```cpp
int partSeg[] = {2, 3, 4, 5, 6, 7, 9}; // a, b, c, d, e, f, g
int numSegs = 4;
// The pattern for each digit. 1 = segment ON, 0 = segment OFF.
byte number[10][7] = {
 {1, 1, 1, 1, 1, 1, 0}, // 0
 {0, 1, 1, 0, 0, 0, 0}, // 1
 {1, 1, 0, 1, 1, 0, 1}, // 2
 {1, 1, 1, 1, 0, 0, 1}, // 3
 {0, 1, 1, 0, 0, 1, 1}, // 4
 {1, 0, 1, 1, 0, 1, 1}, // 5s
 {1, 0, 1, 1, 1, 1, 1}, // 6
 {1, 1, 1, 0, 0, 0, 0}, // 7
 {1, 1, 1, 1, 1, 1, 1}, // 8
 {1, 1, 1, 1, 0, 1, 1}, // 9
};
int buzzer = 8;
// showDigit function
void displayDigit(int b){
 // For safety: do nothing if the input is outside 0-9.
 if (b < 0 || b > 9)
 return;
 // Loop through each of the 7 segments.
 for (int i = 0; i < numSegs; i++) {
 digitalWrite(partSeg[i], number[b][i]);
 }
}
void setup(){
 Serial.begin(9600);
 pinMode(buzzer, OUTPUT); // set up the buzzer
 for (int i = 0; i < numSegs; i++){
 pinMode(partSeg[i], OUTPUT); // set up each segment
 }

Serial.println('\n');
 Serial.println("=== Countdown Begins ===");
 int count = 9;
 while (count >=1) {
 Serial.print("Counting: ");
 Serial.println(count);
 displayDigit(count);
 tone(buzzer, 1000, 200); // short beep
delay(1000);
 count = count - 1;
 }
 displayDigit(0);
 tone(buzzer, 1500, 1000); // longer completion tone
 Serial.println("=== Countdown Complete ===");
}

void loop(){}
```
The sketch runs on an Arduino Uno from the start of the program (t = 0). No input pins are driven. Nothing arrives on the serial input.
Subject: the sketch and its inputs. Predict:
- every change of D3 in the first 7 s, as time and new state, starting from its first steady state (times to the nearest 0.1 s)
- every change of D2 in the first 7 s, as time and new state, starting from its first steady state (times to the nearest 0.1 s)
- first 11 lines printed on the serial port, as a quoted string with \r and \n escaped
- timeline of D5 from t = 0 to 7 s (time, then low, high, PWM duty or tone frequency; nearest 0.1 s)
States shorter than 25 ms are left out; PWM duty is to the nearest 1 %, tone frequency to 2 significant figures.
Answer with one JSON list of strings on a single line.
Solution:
["0 s high; 3 s low; 5 s high", "0 s high; 5 s low; 6 s high", "\"\\n\\r\\n=== Countdown Begins ===\\r\\nCounting: 9\\r\\nCounting: 8\\r\\nCounting: 7\\r\\nCounting: 6\\r\\nCounting: 5\\r\\nCounting: 4\\r\\nCounting: 3\\r\\nCounting: 2\\r\\n\"", "0 s high; 2 s low; 3 s high; 5 s low; 6 s high"]
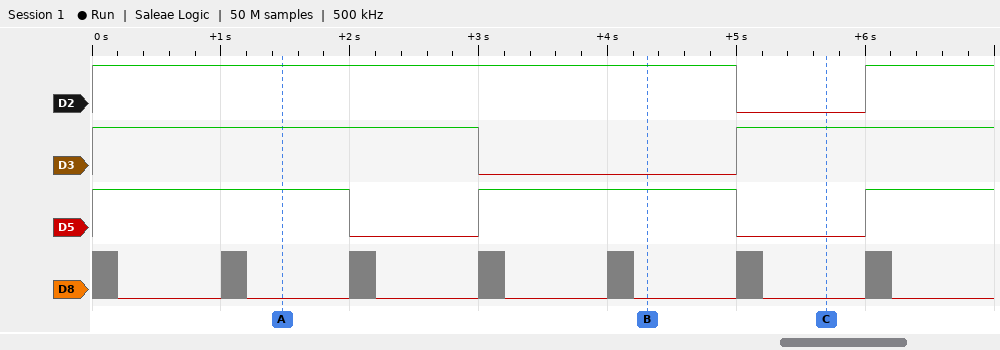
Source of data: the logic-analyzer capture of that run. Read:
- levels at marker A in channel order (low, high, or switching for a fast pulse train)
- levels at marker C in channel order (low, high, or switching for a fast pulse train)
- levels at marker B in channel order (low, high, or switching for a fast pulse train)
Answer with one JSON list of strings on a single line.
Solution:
["D2 high, D3 high, D5 high, D8 low", "D2 low, D3 high, D5 low, D8 low", "D2 high, D3 low, D5 high, D8 low"]
